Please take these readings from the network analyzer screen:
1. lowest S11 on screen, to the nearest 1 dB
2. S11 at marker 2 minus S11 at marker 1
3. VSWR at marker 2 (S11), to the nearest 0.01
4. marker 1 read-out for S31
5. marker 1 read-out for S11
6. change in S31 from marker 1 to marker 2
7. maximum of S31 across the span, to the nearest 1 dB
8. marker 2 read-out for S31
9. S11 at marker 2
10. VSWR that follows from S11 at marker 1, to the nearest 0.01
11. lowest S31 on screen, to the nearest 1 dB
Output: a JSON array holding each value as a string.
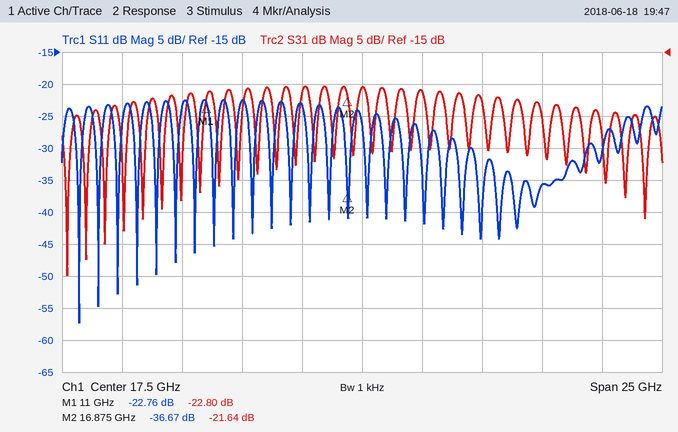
["-57 dB", "-13.91 dB", "1.03", "-22.80 dB", "-22.76 dB", "1.16 dB", "-20 dB", "-21.64 dB", "-36.67 dB", "1.16", "-50 dB"]
